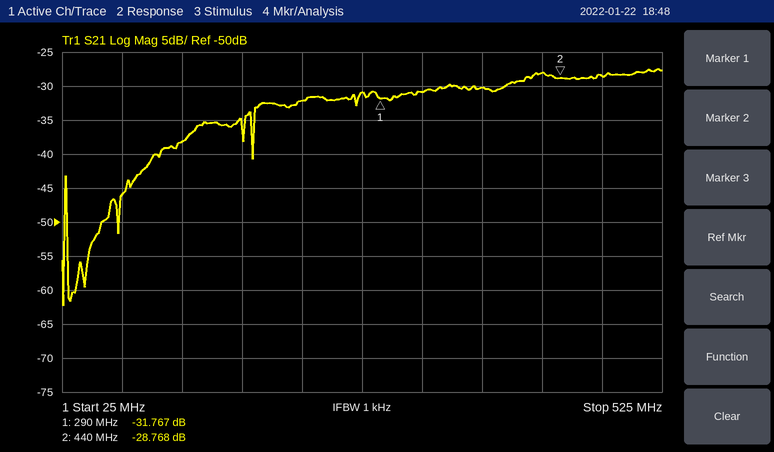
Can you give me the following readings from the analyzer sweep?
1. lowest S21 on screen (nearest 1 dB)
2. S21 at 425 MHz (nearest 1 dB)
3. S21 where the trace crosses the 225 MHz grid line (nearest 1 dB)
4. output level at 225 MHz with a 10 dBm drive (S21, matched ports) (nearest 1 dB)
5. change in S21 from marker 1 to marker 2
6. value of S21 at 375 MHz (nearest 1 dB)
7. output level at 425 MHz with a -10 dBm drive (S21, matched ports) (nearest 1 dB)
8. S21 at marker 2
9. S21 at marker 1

-62 dB
-28 dB
-32 dB
-22 dBm
2.999 dB
-30 dB
-38 dBm
-28.768 dB
-31.767 dB
